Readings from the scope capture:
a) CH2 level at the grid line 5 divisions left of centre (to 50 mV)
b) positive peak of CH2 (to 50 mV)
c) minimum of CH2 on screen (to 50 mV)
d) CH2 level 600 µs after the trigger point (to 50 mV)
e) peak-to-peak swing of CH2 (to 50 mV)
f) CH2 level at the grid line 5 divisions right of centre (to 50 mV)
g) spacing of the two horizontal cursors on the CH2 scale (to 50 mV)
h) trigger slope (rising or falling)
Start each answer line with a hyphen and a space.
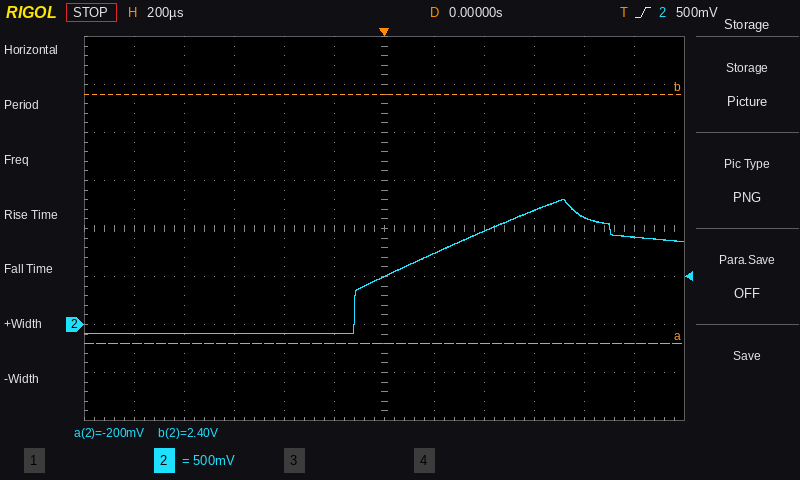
- -100 mV
- 1.30 V
- -100 mV
- 1.20 V
- 1.40 V
- 900 mV
- 2.60 V
- rising
